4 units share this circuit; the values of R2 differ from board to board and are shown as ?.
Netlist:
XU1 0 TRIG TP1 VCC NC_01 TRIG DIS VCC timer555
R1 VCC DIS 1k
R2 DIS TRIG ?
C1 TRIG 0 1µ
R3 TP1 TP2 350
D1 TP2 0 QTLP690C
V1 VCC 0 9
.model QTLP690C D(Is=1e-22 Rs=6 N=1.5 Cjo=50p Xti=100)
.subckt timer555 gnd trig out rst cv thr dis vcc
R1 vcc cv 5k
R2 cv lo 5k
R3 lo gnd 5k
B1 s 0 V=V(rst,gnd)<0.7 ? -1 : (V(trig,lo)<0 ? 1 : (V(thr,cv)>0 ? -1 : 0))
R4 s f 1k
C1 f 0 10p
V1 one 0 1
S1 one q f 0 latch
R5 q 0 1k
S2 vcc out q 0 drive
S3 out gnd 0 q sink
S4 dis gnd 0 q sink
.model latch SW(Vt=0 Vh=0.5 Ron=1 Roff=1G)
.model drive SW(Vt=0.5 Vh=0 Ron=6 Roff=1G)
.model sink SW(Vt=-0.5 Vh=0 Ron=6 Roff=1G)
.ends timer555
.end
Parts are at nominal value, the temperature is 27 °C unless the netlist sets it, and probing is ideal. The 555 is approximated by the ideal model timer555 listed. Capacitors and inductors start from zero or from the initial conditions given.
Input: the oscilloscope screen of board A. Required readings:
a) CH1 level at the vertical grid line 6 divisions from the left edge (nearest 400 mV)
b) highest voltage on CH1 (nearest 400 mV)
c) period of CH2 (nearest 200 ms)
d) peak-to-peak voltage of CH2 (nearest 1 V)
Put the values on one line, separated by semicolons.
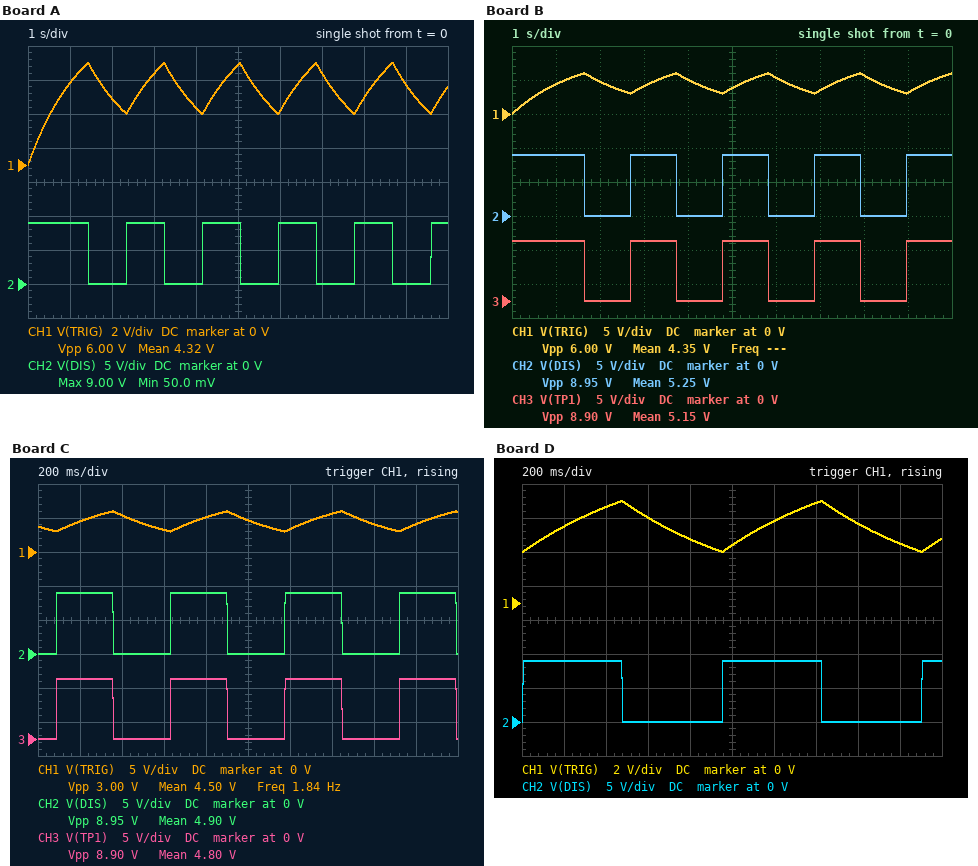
3.2 V; 6.0 V; 1.8 s; 9 V
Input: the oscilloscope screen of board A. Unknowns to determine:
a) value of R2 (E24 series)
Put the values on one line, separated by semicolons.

1.3 MΩ
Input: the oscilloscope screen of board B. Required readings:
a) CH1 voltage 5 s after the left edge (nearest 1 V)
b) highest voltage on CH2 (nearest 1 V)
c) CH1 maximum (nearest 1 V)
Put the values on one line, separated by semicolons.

4 V; 9 V; 6 V
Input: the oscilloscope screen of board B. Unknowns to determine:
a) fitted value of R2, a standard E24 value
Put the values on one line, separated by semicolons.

1.5 MΩ
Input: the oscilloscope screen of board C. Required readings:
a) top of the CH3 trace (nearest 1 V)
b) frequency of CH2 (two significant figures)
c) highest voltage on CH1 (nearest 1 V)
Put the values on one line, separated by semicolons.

9 V; 1.8 Hz; 6 V
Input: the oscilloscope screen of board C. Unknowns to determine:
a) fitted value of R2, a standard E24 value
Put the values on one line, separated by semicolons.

390 kΩ
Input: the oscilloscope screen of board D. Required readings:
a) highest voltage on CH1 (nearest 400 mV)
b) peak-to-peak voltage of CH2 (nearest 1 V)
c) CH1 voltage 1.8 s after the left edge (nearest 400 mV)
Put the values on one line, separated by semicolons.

6.0 V; 9 V; 3.6 V
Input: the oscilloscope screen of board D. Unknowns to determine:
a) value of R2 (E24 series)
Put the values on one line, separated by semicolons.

680 kΩ
